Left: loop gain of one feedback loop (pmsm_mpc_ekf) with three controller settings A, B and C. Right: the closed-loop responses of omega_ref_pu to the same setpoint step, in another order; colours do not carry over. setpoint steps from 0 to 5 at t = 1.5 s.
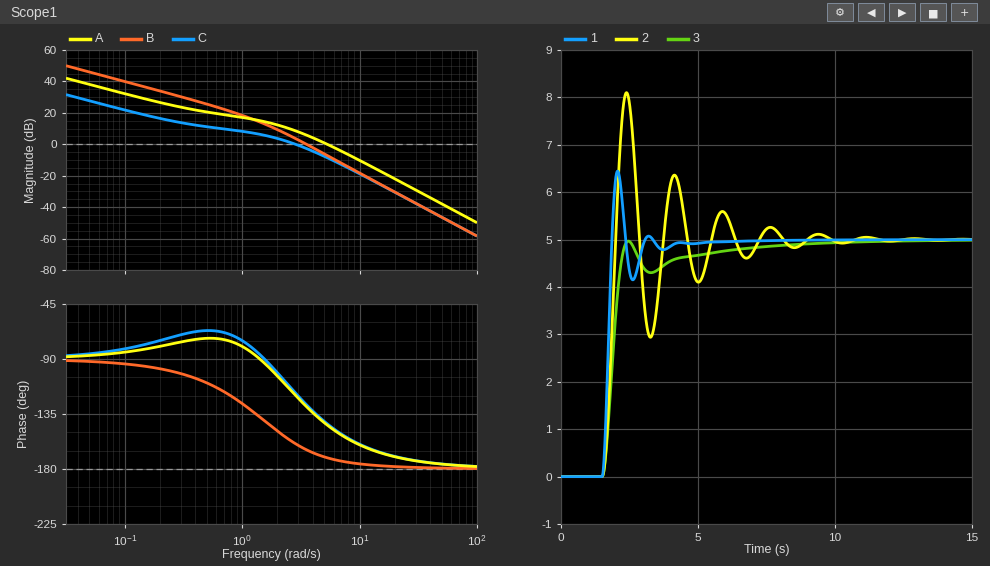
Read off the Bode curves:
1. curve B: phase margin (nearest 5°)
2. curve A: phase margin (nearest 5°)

15°
35°
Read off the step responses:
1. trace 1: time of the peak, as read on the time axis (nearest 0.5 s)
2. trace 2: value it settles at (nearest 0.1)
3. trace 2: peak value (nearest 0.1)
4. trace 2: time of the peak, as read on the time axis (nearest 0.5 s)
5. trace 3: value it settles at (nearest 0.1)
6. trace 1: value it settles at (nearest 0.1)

2.0 s
5.0
8.1
2.5 s
5.0
5.0
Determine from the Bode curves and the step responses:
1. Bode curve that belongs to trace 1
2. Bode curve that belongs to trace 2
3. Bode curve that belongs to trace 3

A
B
C
